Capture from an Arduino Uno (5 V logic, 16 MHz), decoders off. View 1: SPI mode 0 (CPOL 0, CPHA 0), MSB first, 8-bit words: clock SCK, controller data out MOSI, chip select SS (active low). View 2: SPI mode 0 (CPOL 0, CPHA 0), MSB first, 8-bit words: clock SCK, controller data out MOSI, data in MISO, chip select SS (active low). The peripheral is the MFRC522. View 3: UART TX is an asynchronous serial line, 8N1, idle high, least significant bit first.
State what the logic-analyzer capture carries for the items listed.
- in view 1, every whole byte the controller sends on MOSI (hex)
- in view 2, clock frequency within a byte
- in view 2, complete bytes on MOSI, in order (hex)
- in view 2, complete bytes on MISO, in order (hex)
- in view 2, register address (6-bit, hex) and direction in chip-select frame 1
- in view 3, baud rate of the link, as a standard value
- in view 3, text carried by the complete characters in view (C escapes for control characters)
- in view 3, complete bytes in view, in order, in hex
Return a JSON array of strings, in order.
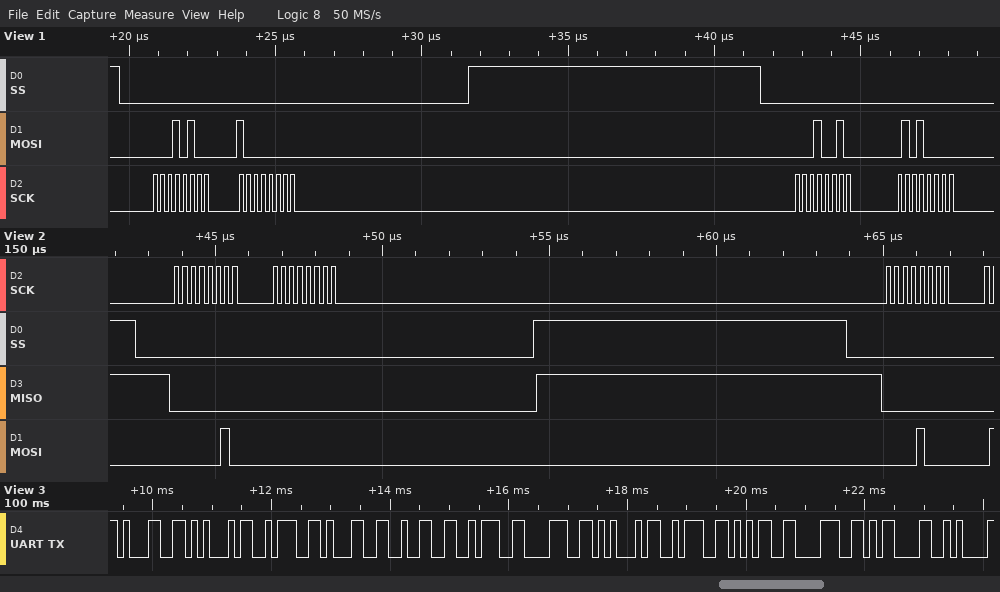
["0x14 0x80 0x12 0x50", "4 MHz", "02 00 08", "00 00 00", "0x01 write", "9600 baud", "\"1E:12:8E:58\\r\\n\"", "31 45 3A 31 32 3A 38 45 3A 35 38 0D 0A"]
